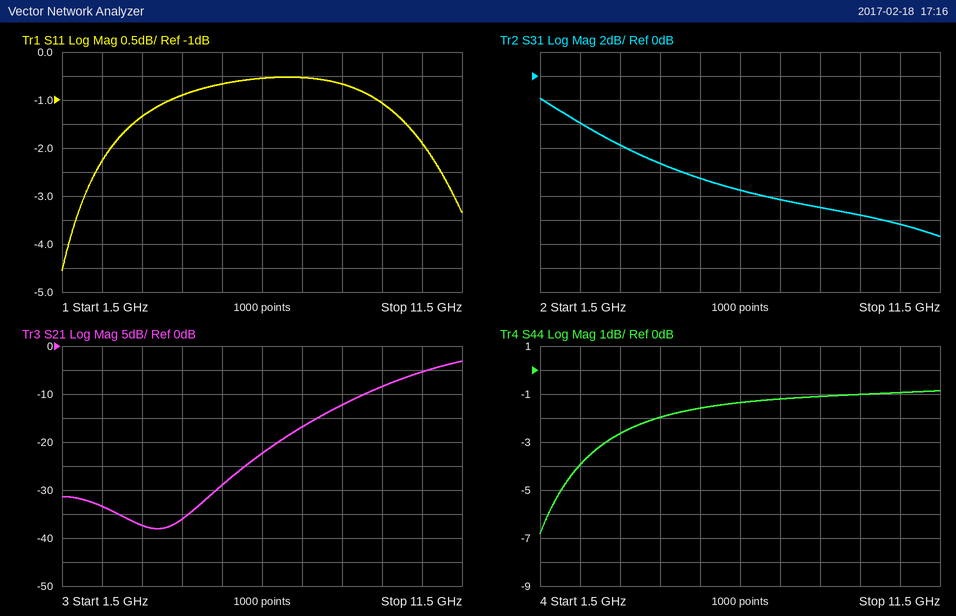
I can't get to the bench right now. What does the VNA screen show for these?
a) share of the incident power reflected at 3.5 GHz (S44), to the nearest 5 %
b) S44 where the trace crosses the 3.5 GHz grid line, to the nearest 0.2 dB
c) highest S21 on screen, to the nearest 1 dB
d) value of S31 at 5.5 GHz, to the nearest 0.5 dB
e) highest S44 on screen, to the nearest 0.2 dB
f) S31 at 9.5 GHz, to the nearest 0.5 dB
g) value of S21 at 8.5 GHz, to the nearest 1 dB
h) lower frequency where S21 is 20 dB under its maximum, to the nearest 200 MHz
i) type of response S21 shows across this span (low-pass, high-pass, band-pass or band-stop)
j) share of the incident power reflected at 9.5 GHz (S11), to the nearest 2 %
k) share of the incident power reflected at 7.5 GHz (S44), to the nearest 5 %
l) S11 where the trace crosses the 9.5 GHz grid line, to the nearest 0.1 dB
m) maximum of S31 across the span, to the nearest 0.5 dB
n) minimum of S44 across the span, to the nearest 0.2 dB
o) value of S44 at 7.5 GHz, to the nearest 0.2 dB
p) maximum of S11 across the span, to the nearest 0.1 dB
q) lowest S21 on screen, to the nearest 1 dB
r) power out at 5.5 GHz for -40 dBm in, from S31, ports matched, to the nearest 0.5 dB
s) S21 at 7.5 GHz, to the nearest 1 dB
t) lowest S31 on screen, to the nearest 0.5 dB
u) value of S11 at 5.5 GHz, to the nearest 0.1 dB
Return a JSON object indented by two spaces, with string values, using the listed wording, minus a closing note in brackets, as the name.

{
  "share of the incident power reflected at 3.5 GHz (S44), to the nearest 5 %": "55 %",
  "S44 where the trace crosses the 3.5 GHz grid line, to the nearest 0.2 dB": "-2.6 dB",
  "highest S21 on screen, to the nearest 1 dB": "-3 dB",
  "value of S31 at 5.5 GHz, to the nearest 0.5 dB": "-8.5 dB",
  "highest S44 on screen, to the nearest 0.2 dB": "-0.8 dB",
  "S31 at 9.5 GHz, to the nearest 0.5 dB": "-11.5 dB",
  "value of S21 at 8.5 GHz, to the nearest 1 dB": "-12 dB",
  "lower frequency where S21 is 20 dB under its maximum, to the nearest 200 MHz": "6.4 GHz",
  "type of response S21 shows across this span": "high-pass",
  "share of the incident power reflected at 9.5 GHz (S11), to the nearest 2 %": "78 %",
  "share of the incident power reflected at 7.5 GHz (S44), to the nearest 5 %": "75 %",
  "S11 where the trace crosses the 9.5 GHz grid line, to the nearest 0.1 dB": "-1.1 dB",
  "maximum of S31 across the span, to the nearest 0.5 dB": "-2.0 dB",
  "minimum of S44 across the span, to the nearest 0.2 dB": "-6.8 dB",
  "value of S44 at 7.5 GHz, to the nearest 0.2 dB": "-1.2 dB",
  "maximum of S11 across the span, to the nearest 0.1 dB": "-0.5 dB",
  "lowest S21 on screen, to the nearest 1 dB": "-38 dB",
  "power out at 5.5 GHz for -40 dBm in, from S31, ports matched, to the nearest 0.5 dB": "-48.5 dBm",
  "S21 at 7.5 GHz, to the nearest 1 dB": "-17 dB",
  "lowest S31 on screen, to the nearest 0.5 dB": "-13.5 dB",
  "value of S11 at 5.5 GHz, to the nearest 0.1 dB": "-0.7 dB"
}
